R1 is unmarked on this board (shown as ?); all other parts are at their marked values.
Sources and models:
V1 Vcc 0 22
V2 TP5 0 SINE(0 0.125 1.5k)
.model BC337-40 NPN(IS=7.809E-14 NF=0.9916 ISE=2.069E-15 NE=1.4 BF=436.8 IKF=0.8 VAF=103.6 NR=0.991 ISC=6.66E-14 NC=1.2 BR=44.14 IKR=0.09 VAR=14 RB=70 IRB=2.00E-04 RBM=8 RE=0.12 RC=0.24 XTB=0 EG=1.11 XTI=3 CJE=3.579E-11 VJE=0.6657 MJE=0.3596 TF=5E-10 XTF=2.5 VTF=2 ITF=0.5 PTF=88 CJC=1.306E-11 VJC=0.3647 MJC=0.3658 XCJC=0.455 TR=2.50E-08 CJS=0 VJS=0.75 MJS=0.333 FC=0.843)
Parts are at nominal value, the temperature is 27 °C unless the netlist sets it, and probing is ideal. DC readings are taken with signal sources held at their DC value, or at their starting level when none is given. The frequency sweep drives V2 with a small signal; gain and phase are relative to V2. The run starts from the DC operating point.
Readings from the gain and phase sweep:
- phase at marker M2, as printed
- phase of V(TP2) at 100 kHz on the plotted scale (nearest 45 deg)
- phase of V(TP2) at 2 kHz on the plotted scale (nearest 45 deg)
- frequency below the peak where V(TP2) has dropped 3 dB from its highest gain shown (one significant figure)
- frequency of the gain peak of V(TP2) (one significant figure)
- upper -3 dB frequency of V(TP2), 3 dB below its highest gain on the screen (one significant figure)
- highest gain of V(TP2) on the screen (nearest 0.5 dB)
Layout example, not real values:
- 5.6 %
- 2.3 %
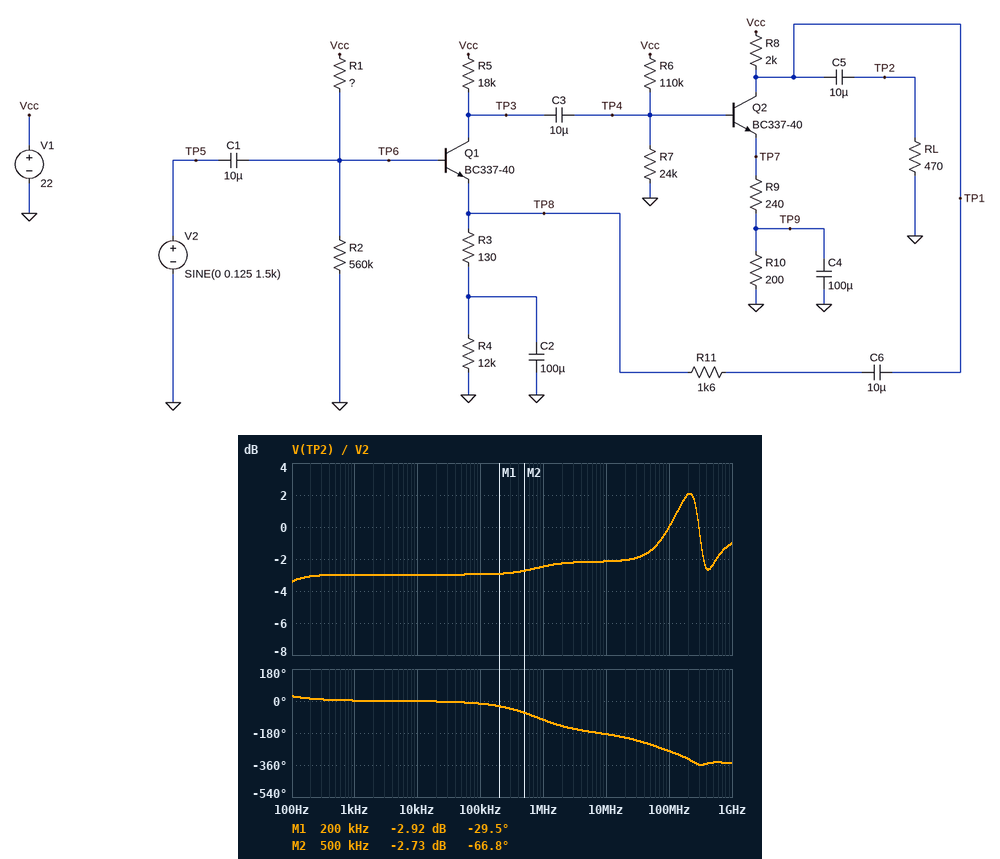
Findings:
- -66.8 deg
- 0 deg
- 0 deg
- 70 MHz
- 200 MHz
- 300 MHz
- 2.0 dB
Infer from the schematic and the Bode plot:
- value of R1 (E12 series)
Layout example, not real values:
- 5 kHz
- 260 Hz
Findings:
- 270 kΩ
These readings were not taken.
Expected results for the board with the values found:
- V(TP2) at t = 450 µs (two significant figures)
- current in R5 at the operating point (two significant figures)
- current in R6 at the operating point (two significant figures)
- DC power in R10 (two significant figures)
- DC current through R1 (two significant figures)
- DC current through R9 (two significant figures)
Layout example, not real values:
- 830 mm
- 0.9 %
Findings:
- -1.1 V
- 720 µA
- 170 µA
- 9.2 mW
- 46 µA
- 6.8 mA
